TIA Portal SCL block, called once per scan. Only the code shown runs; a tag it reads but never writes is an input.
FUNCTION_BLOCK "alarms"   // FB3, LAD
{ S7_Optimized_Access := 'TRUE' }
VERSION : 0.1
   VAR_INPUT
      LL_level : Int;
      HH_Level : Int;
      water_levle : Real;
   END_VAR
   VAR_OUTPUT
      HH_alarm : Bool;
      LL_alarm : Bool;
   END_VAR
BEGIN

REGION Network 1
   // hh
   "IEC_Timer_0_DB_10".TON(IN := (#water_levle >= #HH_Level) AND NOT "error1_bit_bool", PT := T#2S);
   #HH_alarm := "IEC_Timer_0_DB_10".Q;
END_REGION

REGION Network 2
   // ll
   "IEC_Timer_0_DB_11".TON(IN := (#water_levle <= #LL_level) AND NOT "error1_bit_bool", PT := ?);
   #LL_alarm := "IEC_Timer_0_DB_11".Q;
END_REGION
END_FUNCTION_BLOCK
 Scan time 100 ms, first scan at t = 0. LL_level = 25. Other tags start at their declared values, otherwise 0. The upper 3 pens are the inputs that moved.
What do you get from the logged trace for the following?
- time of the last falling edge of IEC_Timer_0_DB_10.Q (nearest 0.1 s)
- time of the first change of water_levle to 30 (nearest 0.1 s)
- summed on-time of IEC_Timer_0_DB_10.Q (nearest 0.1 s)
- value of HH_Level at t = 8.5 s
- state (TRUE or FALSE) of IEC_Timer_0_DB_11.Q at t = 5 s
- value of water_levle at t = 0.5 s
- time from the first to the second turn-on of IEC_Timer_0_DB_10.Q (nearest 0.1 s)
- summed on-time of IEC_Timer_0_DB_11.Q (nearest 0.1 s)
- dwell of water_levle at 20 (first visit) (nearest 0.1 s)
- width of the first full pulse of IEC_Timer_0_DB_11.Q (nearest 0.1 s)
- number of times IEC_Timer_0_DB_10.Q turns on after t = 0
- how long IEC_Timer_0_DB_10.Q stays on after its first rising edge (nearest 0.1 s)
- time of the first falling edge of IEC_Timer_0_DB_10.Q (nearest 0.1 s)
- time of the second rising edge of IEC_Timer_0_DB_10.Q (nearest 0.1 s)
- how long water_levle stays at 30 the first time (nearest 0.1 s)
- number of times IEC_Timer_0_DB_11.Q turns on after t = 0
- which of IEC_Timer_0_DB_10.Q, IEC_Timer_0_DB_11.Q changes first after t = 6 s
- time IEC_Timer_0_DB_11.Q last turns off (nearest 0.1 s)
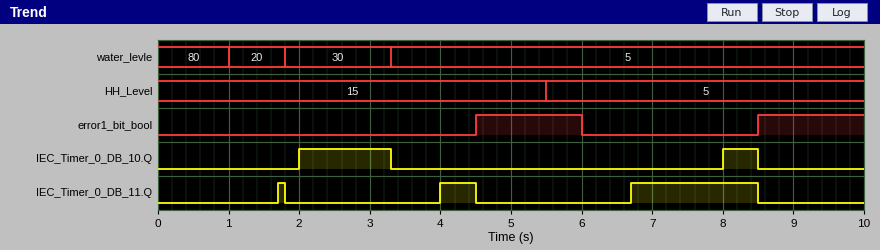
8.5 s
1.8 s
1.8 s
5
FALSE
80
6.0 s
2.4 s
0.8 s
0.1 s
2
1.3 s
3.3 s
8.0 s
1.5 s
3
IEC_Timer_0_DB_11.Q
8.5 s
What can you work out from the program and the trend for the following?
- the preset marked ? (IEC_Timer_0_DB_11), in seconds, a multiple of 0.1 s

0.7 s
